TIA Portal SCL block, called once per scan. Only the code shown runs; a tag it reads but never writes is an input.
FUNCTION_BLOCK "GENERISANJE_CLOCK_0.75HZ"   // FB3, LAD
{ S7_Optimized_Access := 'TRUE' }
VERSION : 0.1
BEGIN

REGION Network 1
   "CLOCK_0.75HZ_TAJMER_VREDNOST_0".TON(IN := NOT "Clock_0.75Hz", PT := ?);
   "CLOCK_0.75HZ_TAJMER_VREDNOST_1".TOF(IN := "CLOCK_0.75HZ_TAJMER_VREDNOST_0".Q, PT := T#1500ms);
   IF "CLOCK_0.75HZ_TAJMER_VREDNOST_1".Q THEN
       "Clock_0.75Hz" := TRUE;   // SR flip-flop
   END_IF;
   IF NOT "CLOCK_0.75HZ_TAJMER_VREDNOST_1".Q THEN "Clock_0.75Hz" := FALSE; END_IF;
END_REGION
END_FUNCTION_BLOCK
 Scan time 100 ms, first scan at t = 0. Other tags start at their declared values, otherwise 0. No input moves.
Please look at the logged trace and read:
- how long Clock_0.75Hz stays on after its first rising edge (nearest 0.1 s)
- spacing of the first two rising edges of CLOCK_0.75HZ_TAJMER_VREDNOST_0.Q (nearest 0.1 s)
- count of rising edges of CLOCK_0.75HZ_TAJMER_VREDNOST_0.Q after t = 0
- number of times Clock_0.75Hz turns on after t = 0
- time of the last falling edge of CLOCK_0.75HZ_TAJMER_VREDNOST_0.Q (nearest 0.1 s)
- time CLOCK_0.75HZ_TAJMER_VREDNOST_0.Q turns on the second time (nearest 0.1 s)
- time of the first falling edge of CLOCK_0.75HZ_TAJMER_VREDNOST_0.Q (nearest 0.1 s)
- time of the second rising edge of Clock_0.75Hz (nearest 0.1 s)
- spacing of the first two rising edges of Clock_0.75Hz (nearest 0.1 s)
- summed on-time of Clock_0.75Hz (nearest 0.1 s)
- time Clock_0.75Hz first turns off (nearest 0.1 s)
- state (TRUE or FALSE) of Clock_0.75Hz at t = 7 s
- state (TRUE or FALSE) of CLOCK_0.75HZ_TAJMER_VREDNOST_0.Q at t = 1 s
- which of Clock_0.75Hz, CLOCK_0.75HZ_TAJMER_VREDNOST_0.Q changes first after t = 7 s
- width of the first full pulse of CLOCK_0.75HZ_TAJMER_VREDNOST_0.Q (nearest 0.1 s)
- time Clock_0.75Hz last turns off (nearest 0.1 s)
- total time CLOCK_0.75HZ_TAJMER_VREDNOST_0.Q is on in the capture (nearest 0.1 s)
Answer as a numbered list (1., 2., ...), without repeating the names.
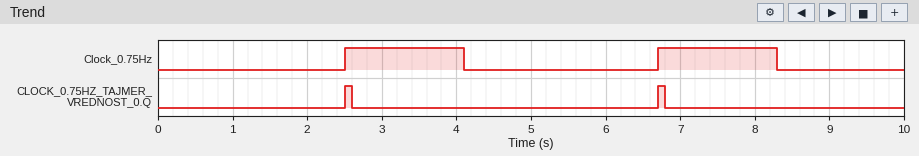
1. 1.6 s
2. 4.2 s
3. 2
4. 2
5. 6.8 s
6. 6.7 s
7. 2.6 s
8. 6.7 s
9. 4.2 s
10. 3.2 s
11. 4.1 s
12. TRUE
13. FALSE
14. Clock_0.75Hz
15. 0.1 s
16. 8.3 s
17. 0.2 s
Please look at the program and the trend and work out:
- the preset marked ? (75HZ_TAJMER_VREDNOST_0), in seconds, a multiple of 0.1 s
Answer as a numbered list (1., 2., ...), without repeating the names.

1. 2.5 s
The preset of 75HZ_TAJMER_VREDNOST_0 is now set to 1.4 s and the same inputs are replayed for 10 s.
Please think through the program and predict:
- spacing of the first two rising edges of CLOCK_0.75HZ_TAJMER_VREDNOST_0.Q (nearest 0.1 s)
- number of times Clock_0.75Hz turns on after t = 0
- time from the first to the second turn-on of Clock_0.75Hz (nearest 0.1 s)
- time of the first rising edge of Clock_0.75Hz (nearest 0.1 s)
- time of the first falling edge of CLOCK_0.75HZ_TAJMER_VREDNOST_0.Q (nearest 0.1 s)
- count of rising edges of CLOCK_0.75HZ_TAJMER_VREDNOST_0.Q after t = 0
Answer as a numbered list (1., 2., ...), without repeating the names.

1. 3.1 s
2. 3
3. 3.1 s
4. 1.4 s
5. 1.5 s
6. 3
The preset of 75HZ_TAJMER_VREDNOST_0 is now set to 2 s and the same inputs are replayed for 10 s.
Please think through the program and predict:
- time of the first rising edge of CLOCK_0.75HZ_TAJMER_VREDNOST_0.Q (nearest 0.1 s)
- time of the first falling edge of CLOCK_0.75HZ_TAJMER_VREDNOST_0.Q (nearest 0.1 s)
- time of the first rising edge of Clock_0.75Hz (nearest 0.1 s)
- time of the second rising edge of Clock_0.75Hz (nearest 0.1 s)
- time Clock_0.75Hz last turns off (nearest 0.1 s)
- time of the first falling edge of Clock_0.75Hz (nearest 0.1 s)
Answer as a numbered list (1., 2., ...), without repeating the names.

1. 2.0 s
2. 2.1 s
3. 2.0 s
4. 5.7 s
5. 7.3 s
6. 3.6 s
